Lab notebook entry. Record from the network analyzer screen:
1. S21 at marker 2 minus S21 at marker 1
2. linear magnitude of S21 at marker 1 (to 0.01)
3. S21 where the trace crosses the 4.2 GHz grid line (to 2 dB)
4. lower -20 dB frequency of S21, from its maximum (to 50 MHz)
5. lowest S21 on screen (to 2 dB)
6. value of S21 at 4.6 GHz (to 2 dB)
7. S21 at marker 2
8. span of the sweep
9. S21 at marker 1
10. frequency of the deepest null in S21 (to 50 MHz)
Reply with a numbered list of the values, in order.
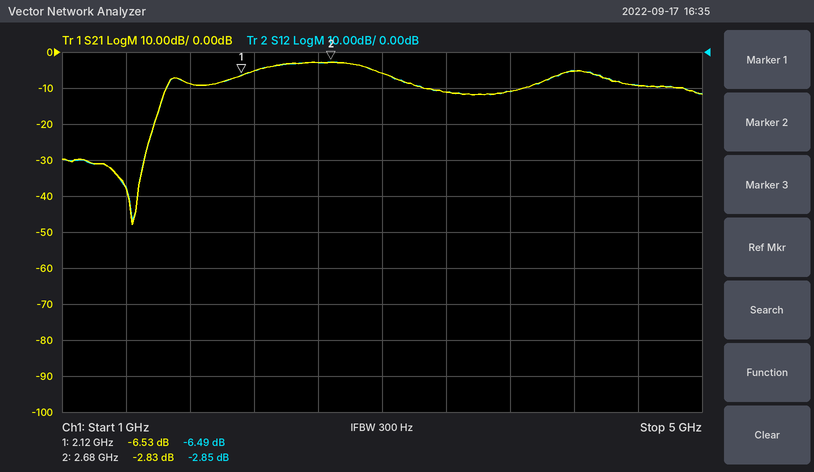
1. 3.70 dB
2. 0.47
3. -6 dB
4. 1.55 GHz
5. -48 dB
6. -10 dB
7. -2.83 dB
8. 4 GHz
9. -6.53 dB
10. 1.45 GHz
